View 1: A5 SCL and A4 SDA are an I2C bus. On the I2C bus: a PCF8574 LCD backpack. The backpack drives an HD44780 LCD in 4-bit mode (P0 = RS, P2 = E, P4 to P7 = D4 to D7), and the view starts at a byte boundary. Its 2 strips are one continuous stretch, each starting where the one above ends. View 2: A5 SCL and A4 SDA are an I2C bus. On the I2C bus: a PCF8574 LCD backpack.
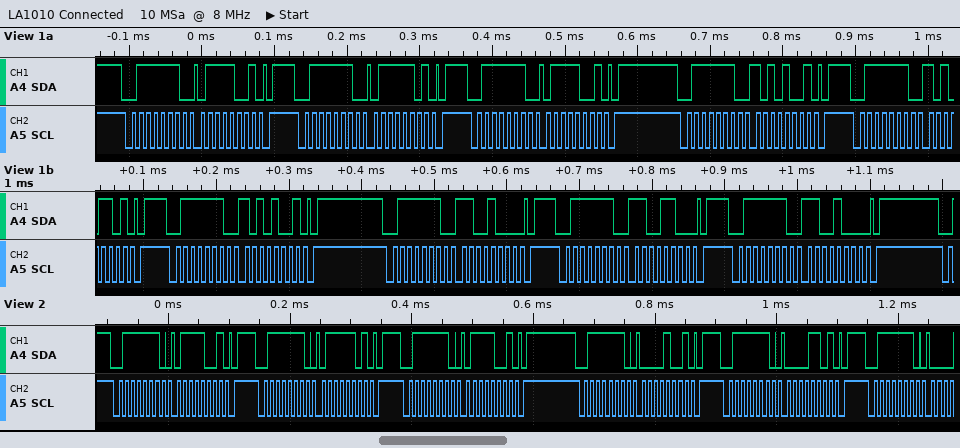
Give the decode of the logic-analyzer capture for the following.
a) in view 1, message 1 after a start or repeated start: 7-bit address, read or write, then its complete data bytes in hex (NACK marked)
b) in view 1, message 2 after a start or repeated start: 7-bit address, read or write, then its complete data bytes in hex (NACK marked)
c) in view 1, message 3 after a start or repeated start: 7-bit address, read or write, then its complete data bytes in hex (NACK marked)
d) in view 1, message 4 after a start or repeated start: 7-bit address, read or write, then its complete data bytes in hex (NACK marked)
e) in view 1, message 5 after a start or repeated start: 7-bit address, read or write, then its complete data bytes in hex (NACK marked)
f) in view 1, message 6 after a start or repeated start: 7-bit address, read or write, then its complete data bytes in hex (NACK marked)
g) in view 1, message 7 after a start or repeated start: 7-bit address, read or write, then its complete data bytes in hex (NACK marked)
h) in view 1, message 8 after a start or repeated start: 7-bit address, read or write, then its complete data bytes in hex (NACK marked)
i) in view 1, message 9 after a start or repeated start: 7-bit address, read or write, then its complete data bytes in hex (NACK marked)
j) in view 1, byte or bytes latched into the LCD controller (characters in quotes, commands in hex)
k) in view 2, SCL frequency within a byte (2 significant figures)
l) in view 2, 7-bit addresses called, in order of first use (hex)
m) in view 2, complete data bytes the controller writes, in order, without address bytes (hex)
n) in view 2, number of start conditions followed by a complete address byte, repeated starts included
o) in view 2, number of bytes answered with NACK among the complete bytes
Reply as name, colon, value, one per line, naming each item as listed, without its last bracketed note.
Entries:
in view 1, message 1 after a start or repeated start: 7-bit address, read or write, then its complete data bytes in hex: 0x3F write: 79
in view 1, message 2 after a start or repeated start: 7-bit address, read or write, then its complete data bytes in hex: 0x3F write: 7D
in view 1, message 3 after a start or repeated start: 7-bit address, read or write, then its complete data bytes in hex: 0x3F write: 79
in view 1, message 4 after a start or repeated start: 7-bit address, read or write, then its complete data bytes in hex: 0x3F write: A9
in view 1, message 5 after a start or repeated start: 7-bit address, read or write, then its complete data bytes in hex: 0x3F write: AD
in view 1, message 6 after a start or repeated start: 7-bit address, read or write, then its complete data bytes in hex: 0x3F write: A9
in view 1, message 7 after a start or repeated start: 7-bit address, read or write, then its complete data bytes in hex: 0x3F write: C8
in view 1, message 8 after a start or repeated start: 7-bit address, read or write, then its complete data bytes in hex: 0x3F write: CC
in view 1, message 9 after a start or repeated start: 7-bit address, read or write, then its complete data bytes in hex: 0x3F write: C8
in view 1, byte or bytes latched into the LCD controller: 'z'
in view 2, SCL frequency within a byte: 100 kHz
in view 2, 7-bit addresses called, in order of first use: 0x3F
in view 2, complete data bytes the controller writes, in order, without address bytes: 79 7D 79 09 0D
in view 2, number of start conditions followed by a complete address byte, repeated starts included: 6
in view 2, number of bytes answered with NACK among the complete bytes: 0
